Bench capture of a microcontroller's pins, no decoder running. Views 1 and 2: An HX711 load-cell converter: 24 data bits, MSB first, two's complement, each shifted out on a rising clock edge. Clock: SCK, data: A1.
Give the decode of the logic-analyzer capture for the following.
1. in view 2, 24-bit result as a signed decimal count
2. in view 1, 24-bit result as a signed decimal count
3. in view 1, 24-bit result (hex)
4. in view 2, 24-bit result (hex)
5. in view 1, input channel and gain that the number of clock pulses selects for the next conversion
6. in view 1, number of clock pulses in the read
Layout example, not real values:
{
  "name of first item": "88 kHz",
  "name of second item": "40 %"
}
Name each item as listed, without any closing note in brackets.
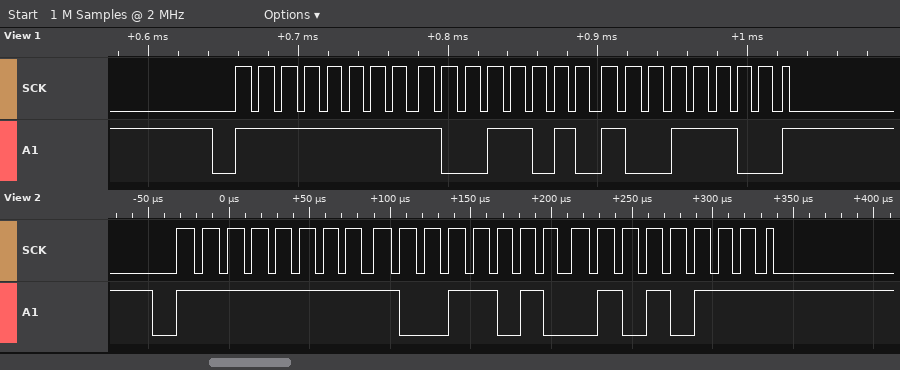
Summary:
{
  "in view 2, 24-bit result as a signed decimal count": "-26025",
  "in view 1, 24-bit result as a signed decimal count": "-25956",
  "in view 1, 24-bit result": "0xFF9A9C",
  "in view 2, 24-bit result": "0xFF9A57",
  "in view 1, input channel and gain that the number of clock pulses selects for the next conversion": "channel A, gain 128",
  "in view 1, number of clock pulses in the read": "25"
}
